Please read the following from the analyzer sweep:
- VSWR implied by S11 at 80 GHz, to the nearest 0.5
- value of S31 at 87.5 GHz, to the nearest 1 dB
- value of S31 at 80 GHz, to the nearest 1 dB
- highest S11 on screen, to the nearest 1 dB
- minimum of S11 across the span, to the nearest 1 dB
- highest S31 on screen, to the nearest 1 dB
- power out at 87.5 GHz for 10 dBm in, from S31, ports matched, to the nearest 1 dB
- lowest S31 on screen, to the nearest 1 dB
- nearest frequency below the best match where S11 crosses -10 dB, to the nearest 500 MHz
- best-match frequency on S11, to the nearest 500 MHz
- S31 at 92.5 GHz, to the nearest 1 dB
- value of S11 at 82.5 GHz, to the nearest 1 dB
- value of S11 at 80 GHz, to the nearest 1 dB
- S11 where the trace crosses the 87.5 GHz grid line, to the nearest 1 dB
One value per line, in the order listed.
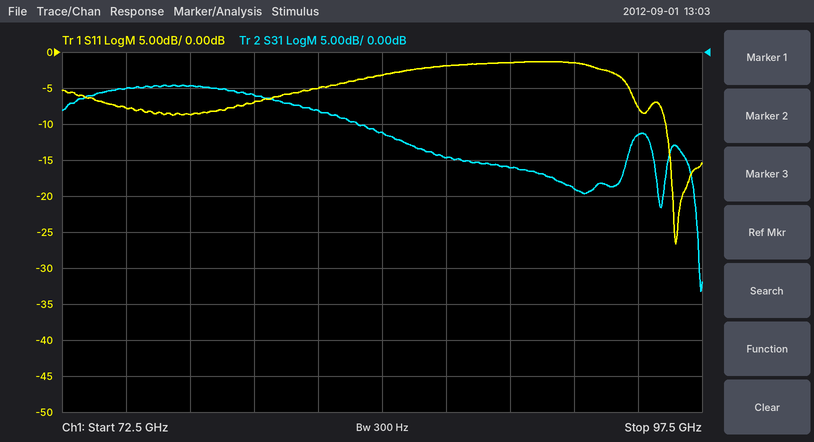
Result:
2.5
-15 dB
-6 dB
-1 dB
-27 dB
-5 dB
-5 dBm
-33 dB
96.0 GHz
96.5 GHz
-19 dB
-5 dB
-7 dB
-2 dB
